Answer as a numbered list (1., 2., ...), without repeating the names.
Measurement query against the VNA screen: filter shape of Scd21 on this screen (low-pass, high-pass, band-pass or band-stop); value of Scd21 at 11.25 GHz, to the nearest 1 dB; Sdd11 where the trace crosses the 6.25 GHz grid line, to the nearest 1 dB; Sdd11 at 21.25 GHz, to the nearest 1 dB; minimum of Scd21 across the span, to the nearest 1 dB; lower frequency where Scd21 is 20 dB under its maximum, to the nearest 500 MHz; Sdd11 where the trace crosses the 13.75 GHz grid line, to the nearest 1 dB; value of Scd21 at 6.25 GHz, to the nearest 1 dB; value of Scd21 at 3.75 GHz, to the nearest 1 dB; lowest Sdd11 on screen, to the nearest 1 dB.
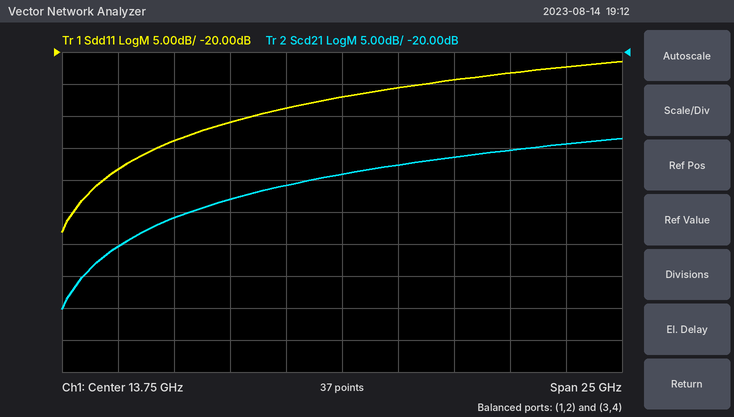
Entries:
1. high-pass
2. -41 dB
3. -34 dB
4. -23 dB
5. -60 dB
6. 2.5 GHz
7. -27 dB
8. -46 dB
9. -50 dB
10. -48 dB
